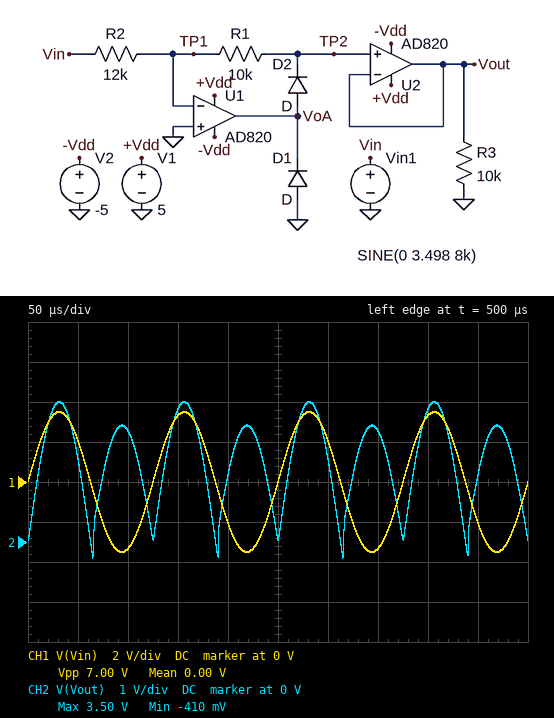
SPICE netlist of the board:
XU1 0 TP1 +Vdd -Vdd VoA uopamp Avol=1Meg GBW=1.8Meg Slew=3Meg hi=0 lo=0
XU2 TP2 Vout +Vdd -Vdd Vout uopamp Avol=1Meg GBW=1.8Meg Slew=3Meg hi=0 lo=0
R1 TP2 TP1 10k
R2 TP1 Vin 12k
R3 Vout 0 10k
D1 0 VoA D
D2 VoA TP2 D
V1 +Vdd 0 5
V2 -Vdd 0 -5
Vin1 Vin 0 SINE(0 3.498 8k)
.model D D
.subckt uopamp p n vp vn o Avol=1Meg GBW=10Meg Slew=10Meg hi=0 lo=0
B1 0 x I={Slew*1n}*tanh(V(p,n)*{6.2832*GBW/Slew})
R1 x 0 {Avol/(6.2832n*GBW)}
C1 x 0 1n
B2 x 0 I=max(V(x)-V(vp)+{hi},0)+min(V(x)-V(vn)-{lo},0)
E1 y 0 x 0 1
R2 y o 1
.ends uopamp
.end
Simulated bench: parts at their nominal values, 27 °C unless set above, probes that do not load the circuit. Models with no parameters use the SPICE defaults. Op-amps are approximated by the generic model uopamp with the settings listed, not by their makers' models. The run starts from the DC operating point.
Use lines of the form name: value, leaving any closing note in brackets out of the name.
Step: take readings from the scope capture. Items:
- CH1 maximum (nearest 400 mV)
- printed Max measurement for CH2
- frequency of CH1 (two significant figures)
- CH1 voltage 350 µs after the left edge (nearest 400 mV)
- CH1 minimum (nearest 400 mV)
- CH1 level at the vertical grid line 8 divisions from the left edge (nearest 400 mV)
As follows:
CH1 maximum: 3.6 V
printed Max measurement for CH2: 3.50 V
frequency of CH1: 8.0 kHz
CH1 voltage 350 µs after the left edge: -3.2 V
CH1 minimum: -3.6 V
CH1 level at the vertical grid line 8 divisions from the left edge: 3.2 V
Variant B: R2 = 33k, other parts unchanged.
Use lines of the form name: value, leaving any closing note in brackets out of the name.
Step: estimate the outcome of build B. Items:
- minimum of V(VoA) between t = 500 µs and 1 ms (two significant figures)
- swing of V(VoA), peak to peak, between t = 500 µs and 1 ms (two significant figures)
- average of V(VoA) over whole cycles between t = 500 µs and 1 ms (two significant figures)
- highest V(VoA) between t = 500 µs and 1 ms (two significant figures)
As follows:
minimum of V(VoA) between t = 500 µs and 1 ms: -870 mV
swing of V(VoA), peak to peak, between t = 500 µs and 1 ms: 2.5 V
average of V(VoA) over whole cycles between t = 500 µs and 1 ms: 170 mV
highest V(VoA) between t = 500 µs and 1 ms: 1.7 V
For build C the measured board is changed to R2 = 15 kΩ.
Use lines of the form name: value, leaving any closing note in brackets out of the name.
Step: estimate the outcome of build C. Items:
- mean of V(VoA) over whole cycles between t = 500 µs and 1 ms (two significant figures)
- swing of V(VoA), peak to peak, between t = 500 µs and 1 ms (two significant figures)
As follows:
mean of V(VoA) over whole cycles between t = 500 µs and 1 ms: 580 mV
swing of V(VoA), peak to peak, between t = 500 µs and 1 ms: 3.8 V
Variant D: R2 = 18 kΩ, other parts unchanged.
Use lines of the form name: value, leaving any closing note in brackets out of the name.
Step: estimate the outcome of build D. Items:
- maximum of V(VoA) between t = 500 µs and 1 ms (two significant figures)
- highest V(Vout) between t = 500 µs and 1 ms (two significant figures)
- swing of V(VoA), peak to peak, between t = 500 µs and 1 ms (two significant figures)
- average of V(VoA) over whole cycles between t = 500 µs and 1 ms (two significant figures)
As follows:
maximum of V(VoA) between t = 500 µs and 1 ms: 2.6 V
highest V(Vout) between t = 500 µs and 1 ms: 3.5 V
swing of V(VoA), peak to peak, between t = 500 µs and 1 ms: 3.4 V
average of V(VoA) over whole cycles between t = 500 µs and 1 ms: 460 mV
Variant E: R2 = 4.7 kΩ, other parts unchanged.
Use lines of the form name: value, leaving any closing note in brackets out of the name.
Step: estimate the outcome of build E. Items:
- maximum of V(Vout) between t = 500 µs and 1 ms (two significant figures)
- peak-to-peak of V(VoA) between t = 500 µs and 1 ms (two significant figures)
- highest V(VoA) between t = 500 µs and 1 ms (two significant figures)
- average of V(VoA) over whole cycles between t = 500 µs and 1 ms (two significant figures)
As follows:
maximum of V(Vout) between t = 500 µs and 1 ms: 4.4 V
peak-to-peak of V(VoA) between t = 500 µs and 1 ms: 5.9 V
highest V(VoA) between t = 500 µs and 1 ms: 5.0 V
average of V(VoA) over whole cycles between t = 500 µs and 1 ms: 1.6 V
